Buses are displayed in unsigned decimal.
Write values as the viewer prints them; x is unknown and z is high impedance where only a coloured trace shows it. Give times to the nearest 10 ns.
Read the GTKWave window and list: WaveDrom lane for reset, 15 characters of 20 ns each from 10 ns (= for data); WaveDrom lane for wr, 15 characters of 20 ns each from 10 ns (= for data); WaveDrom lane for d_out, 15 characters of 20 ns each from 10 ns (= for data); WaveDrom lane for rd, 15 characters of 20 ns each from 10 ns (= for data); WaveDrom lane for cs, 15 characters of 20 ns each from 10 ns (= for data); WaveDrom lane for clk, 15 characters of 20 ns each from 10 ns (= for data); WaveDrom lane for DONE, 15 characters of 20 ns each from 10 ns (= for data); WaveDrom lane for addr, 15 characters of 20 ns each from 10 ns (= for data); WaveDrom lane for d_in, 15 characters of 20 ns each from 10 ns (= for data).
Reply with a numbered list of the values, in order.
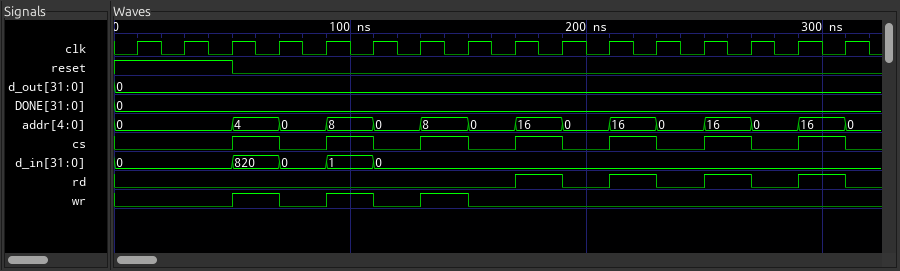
1. {name: 'reset', wave: '1.0............'}
2. {name: 'wr', wave: '0.101010.......'}
3. {name: 'd_out', wave: '=..............', data: '0'}
4. {name: 'rd', wave: '0.......1010101'}
5. {name: 'cs', wave: '0.1010101010101'}
6. {name: 'clk', wave: 'p..............'}
7. {name: 'DONE', wave: '=..............', data: '0'}
8. {name: 'addr', wave: '=.=============', data: '0 4 0 8 0 8 0 16 0 16 0 16 0 16'}
9. {name: 'd_in', wave: '=.====.........', data: '0 820 0 1 0'}
